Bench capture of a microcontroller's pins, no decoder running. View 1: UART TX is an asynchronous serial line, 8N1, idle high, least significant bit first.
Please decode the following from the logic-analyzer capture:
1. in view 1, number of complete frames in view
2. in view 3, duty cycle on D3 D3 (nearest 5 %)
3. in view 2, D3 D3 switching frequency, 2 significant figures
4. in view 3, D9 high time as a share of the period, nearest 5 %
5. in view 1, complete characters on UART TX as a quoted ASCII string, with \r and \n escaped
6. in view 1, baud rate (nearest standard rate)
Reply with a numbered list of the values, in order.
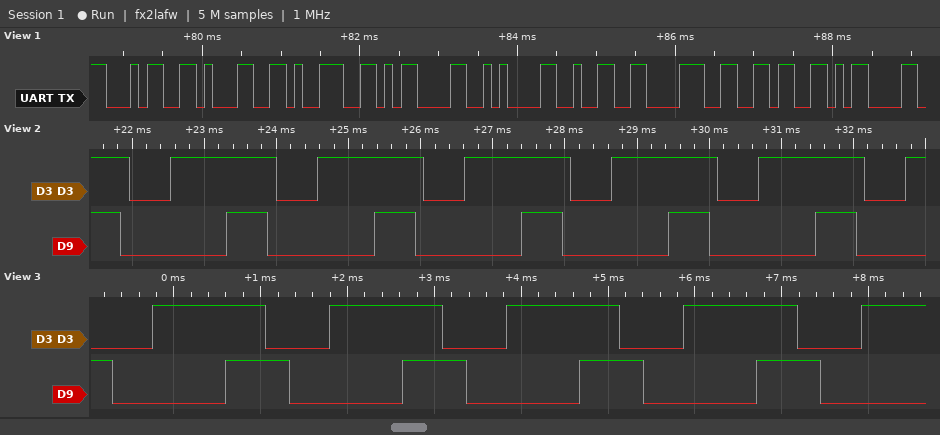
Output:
1. 9
2. 65 %
3. 490 Hz
4. 35 %
5. "419\r\n286\r"
6. 9600 baud
